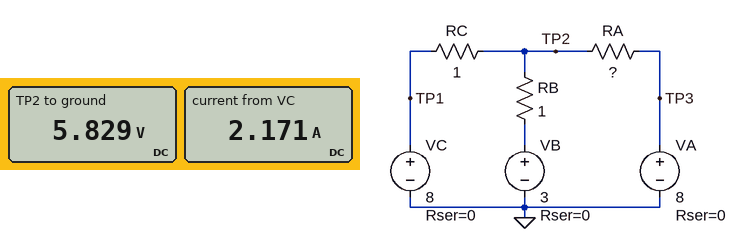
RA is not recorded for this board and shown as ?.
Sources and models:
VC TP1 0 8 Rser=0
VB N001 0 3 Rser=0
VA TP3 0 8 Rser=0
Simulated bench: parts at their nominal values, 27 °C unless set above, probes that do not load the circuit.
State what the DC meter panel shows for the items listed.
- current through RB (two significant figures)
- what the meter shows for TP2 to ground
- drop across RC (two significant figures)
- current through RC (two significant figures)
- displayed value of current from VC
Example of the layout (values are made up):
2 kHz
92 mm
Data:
2.8 A
5.829 V
2.2 V
2.2 A
2.171 A
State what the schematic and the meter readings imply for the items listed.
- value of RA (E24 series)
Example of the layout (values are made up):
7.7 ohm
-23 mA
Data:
3.3 Ω
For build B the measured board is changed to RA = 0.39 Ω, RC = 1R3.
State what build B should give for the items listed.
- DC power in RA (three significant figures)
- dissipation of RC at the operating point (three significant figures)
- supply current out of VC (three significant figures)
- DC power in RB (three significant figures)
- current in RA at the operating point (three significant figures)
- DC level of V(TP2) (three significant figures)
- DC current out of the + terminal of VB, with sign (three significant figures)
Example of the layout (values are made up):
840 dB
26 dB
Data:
3.41 W
1.02 W
888 mA
14.8 W
2.96 A
6.85 V
-3.85 A
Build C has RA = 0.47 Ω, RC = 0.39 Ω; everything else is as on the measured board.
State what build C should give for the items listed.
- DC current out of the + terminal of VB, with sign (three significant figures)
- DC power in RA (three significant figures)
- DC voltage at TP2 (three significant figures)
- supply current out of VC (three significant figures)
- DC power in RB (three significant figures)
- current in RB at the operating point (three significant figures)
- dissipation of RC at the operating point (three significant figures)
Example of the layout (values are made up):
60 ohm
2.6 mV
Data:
-4.12 A
1.64 W
7.12 V
2.25 A
17.0 W
4.12 A
1.98 W
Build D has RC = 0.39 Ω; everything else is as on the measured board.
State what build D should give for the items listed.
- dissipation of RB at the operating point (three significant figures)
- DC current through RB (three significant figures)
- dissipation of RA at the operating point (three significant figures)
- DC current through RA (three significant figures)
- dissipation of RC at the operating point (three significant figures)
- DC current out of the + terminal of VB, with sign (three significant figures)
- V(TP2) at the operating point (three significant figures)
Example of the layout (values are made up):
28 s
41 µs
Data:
13.7 W
3.71 A
507 mW
392 mA
4.29 W
-3.71 A
6.71 V
